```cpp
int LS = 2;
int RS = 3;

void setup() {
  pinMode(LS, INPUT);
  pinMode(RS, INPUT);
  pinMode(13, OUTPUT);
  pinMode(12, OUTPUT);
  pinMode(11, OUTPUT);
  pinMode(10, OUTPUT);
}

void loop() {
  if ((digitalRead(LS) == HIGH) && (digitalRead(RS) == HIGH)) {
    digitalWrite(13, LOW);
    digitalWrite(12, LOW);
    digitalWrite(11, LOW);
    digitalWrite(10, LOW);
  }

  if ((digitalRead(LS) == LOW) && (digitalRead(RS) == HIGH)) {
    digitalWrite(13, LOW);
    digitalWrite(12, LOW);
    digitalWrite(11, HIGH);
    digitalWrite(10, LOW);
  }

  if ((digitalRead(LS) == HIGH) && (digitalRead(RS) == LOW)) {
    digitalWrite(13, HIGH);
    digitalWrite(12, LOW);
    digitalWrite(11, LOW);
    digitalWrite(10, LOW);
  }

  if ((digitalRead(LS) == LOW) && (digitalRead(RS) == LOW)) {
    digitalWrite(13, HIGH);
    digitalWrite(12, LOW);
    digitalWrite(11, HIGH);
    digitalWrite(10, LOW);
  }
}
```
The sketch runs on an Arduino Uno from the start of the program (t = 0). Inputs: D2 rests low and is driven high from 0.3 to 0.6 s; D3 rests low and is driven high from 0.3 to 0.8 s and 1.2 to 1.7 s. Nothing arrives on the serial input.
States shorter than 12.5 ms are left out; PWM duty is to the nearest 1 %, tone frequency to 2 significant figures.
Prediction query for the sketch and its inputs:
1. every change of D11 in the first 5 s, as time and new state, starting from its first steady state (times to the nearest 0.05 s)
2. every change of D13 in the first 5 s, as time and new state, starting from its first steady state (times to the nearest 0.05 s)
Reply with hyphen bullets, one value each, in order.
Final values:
- 0 s high; 0.3 s low; 0.6 s high
- 0 s high; 0.3 s low; 0.8 s high; 1.2 s low; 1.7 s high
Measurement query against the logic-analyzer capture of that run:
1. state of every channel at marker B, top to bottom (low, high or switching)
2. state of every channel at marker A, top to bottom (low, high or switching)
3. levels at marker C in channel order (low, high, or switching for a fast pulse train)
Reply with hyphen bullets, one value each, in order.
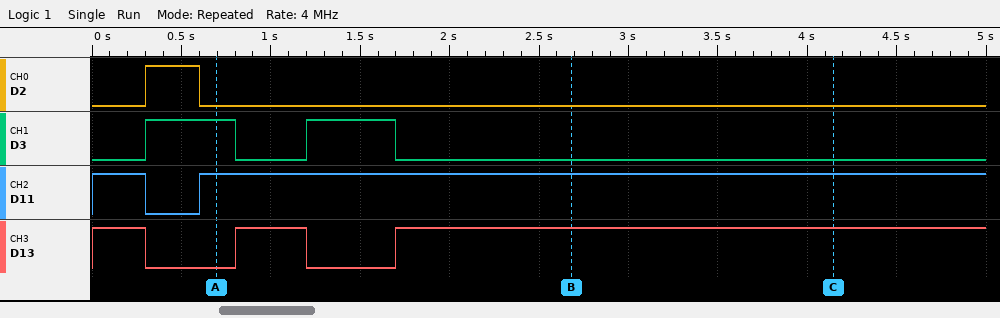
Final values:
- D2 low, D3 low, D11 high, D13 high
- D2 low, D3 high, D11 high, D13 low
- D2 low, D3 low, D11 high, D13 high
